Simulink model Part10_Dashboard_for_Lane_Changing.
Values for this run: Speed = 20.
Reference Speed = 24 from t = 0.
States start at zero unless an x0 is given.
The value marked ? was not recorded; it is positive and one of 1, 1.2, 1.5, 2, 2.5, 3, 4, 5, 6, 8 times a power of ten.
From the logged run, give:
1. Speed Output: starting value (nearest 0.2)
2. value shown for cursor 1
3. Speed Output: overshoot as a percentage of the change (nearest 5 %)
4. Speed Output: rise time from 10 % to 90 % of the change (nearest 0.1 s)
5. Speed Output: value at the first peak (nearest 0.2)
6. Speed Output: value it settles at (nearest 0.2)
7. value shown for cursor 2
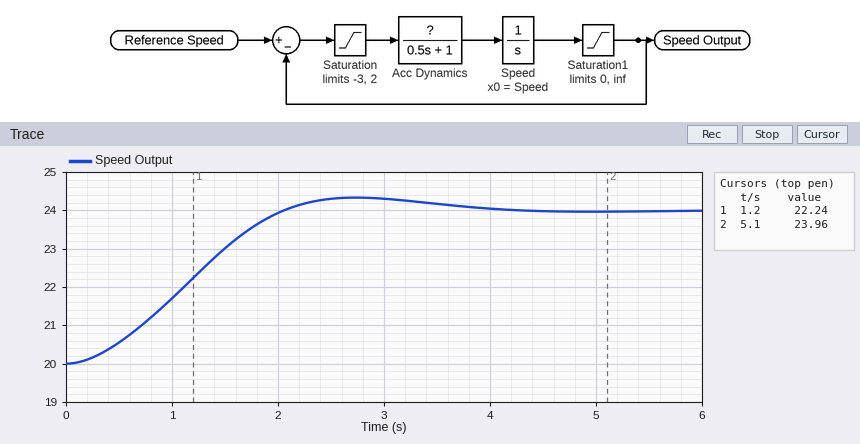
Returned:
20.0
22.24
10 %
1.4 s
24.4
24.0
23.96
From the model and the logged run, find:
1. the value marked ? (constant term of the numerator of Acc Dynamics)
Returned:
1.5
